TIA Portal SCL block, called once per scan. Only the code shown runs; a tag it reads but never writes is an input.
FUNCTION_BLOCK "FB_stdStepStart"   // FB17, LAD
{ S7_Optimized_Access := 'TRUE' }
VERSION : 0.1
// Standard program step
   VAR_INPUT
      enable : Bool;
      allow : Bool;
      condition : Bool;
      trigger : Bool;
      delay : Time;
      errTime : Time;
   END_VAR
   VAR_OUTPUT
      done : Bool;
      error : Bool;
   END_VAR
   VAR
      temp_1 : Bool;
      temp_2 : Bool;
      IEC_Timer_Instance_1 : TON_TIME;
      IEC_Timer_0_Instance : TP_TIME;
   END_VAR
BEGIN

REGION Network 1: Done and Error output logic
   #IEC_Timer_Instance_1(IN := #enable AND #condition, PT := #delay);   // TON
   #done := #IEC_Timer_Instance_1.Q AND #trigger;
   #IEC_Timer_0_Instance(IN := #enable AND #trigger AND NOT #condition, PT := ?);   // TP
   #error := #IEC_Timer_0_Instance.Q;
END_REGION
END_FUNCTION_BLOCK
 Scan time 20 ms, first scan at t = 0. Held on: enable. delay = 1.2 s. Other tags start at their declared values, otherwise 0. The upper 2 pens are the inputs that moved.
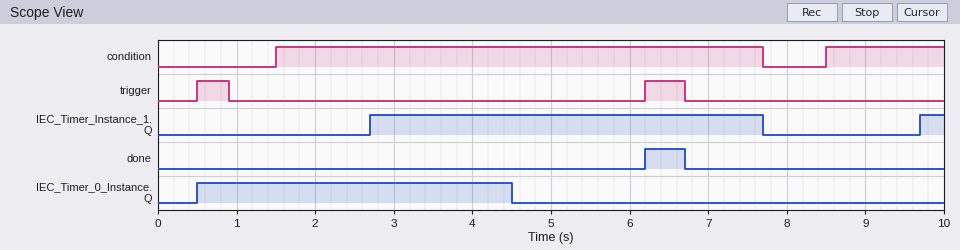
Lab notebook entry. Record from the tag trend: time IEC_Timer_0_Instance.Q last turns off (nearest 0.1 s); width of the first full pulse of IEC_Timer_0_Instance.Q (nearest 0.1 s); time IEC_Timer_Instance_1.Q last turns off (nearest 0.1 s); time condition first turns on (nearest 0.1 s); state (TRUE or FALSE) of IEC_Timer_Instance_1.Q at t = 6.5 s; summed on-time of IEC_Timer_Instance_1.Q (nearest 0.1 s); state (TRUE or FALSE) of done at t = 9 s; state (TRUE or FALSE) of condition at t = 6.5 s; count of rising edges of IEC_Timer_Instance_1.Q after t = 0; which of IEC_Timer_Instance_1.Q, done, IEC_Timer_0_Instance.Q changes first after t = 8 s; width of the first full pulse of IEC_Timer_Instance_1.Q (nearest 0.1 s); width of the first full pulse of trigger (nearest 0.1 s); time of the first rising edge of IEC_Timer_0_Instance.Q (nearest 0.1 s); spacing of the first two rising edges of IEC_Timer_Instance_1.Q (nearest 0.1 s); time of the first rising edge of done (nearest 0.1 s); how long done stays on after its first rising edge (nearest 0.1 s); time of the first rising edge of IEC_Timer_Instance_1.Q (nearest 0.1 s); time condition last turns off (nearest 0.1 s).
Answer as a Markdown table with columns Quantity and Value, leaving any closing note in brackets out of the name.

| Quantity | Value |
|---|---|
| time IEC_Timer_0_Instance.Q last turns off | 4.5 s |
| width of the first full pulse of IEC_Timer_0_Instance.Q | 4.0 s |
| time IEC_Timer_Instance_1.Q last turns off | 7.7 s |
| time condition first turns on | 1.5 s |
| state (TRUE or FALSE) of IEC_Timer_Instance_1.Q at t = 6.5 s | TRUE |
| summed on-time of IEC_Timer_Instance_1.Q | 5.3 s |
| state (TRUE or FALSE) of done at t = 9 s | FALSE |
| state (TRUE or FALSE) of condition at t = 6.5 s | TRUE |
| count of rising edges of IEC_Timer_Instance_1.Q after t = 0 | 2 |
| which of IEC_Timer_Instance_1.Q, done, IEC_Timer_0_Instance.Q changes first after t = 8 s | IEC_Timer_Instance_1.Q |
| width of the first full pulse of IEC_Timer_Instance_1.Q | 5.0 s |
| width of the first full pulse of trigger | 0.4 s |
| time of the first rising edge of IEC_Timer_0_Instance.Q | 0.5 s |
| spacing of the first two rising edges of IEC_Timer_Instance_1.Q | 7.0 s |
| time of the first rising edge of done | 6.2 s |
| how long done stays on after its first rising edge | 0.5 s |
| time of the first rising edge of IEC_Timer_Instance_1.Q | 2.7 s |
| time condition last turns off | 7.7 s |
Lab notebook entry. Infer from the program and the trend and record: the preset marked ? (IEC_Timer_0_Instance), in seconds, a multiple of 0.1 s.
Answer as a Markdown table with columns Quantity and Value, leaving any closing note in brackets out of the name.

| Quantity | Value |
|---|---|
| the preset marked ? (IEC_Timer_0_Instance), in seconds, a multiple of 0.1 s | 4.0 s |
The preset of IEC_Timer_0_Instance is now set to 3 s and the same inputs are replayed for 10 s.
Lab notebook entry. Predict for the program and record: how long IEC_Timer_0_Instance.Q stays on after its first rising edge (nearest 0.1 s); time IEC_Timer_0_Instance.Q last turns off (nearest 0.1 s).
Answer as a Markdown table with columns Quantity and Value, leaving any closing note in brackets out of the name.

| Quantity | Value |
|---|---|
| how long IEC_Timer_0_Instance.Q stays on after its first rising edge | 3.0 s |
| time IEC_Timer_0_Instance.Q last turns off | 3.5 s |
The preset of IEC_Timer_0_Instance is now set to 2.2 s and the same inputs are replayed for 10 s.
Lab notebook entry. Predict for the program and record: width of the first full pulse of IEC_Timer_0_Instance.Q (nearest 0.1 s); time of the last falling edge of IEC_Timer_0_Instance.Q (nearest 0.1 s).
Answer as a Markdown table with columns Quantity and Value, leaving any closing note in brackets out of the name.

| Quantity | Value |
|---|---|
| width of the first full pulse of IEC_Timer_0_Instance.Q | 2.2 s |
| time of the last falling edge of IEC_Timer_0_Instance.Q | 2.7 s |
